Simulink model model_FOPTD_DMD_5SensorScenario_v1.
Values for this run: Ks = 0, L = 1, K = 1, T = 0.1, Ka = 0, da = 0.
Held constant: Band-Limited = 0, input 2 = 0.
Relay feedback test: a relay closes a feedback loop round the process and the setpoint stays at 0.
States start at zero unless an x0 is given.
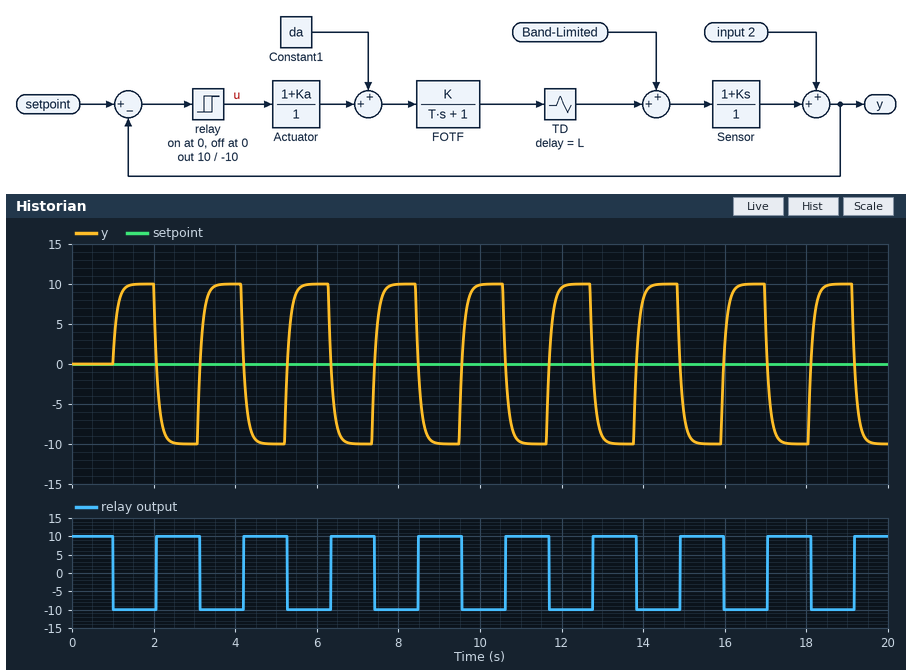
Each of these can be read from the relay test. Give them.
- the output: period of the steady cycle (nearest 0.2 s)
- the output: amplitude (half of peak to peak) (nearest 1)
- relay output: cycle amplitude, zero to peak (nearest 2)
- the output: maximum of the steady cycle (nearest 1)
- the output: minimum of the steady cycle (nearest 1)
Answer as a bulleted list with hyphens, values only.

- 2.2 s
- 10
- 10
- 10
- -10
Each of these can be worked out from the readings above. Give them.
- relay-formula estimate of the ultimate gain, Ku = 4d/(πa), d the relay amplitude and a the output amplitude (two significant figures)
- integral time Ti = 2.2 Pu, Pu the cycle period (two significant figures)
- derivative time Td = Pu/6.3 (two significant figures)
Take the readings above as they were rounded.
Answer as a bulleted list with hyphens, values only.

- 1.3
- 4.8 s
- 0.35 s
